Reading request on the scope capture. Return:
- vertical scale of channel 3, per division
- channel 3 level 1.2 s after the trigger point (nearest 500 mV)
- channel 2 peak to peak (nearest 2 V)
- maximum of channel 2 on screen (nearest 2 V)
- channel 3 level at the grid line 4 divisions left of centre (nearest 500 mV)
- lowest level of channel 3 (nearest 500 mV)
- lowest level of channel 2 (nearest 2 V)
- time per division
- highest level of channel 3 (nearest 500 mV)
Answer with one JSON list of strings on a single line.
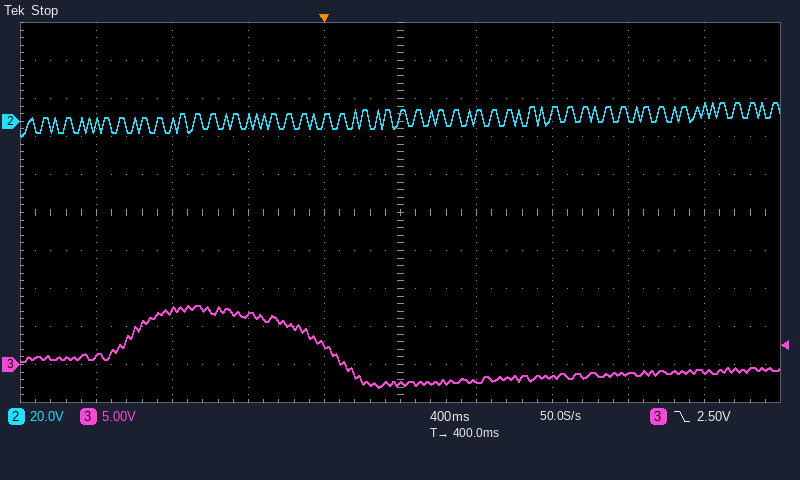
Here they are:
["5 V", "-1.5 V", "18 V", "10 V", "1.0 V", "-3.0 V", "-8 V", "400 ms", "8.0 V"]
